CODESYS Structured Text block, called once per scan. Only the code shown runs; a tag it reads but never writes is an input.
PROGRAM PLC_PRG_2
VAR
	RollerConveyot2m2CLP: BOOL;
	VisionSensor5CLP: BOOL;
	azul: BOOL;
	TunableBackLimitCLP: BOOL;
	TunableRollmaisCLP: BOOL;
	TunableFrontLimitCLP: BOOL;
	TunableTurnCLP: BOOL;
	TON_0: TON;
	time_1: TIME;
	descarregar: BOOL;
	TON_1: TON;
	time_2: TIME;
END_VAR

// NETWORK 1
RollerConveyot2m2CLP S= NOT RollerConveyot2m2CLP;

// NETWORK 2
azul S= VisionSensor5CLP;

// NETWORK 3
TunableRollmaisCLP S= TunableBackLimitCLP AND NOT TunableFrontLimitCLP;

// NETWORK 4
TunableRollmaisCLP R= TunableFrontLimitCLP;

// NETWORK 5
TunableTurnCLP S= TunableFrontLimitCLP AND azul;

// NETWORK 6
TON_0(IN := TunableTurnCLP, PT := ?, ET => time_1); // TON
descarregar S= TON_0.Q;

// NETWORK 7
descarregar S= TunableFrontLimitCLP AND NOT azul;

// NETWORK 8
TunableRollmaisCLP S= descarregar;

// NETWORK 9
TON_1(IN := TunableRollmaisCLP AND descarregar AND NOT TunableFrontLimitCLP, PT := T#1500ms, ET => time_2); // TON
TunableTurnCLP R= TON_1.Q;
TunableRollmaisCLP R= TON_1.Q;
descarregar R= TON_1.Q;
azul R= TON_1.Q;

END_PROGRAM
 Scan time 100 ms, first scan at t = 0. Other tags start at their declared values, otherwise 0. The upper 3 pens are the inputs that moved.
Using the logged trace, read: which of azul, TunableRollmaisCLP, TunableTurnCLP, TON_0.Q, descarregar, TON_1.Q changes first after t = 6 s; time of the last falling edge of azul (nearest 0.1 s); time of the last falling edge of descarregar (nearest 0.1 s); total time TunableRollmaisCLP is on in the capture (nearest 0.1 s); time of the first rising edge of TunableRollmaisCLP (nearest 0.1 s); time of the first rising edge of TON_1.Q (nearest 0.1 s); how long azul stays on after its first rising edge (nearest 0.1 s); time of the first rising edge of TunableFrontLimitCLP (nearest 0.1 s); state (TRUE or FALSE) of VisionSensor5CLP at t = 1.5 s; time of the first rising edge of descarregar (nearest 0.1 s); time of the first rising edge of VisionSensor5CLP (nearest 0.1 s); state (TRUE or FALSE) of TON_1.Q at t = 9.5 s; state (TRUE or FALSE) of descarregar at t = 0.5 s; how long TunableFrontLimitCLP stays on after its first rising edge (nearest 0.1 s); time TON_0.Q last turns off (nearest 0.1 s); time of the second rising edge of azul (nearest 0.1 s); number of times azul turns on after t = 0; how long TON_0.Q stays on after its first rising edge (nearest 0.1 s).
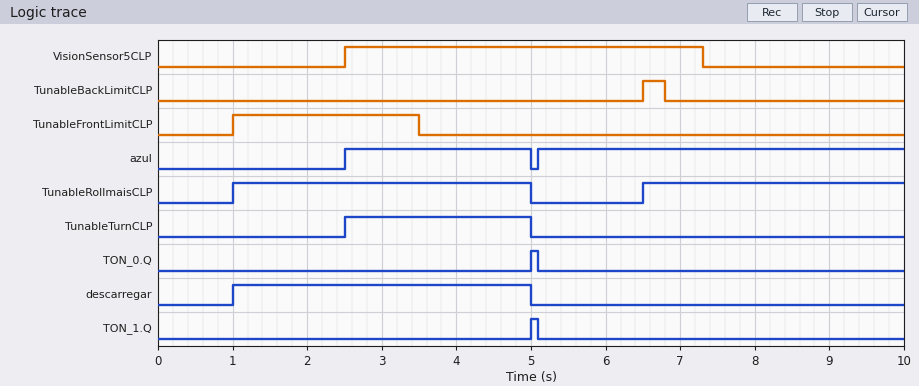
TunableRollmaisCLP
5.0 s
5.0 s
7.5 s
1.0 s
5.0 s
2.5 s
1.0 s
FALSE
1.0 s
2.5 s
FALSE
FALSE
2.5 s
5.1 s
5.1 s
2
0.1 s
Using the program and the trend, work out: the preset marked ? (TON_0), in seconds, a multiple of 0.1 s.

2.5 s
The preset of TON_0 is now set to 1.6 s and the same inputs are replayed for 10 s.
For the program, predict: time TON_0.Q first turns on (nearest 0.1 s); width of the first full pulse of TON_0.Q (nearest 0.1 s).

4.1 s
1.0 s
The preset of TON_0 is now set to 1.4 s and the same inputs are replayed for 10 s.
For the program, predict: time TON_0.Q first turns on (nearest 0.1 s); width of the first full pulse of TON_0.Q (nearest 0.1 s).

3.9 s
1.2 s
